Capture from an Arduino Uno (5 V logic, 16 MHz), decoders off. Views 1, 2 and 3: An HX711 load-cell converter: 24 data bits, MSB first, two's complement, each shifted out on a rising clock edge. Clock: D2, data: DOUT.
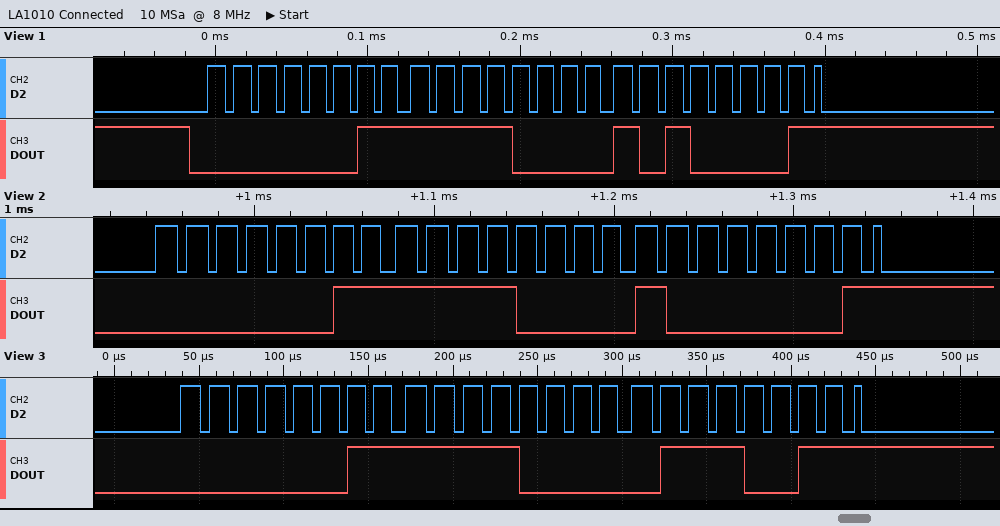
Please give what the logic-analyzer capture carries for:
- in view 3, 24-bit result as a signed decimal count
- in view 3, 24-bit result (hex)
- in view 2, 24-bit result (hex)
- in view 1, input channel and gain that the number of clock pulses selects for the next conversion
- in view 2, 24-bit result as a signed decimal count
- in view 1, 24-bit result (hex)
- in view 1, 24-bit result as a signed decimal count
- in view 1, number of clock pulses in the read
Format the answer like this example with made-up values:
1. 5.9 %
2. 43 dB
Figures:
1. 258163
2. 0x03F073
3. 0x03F081
4. channel A, gain 128
5. 258177
6. 0x03F0A1
7. 258209
8. 25
